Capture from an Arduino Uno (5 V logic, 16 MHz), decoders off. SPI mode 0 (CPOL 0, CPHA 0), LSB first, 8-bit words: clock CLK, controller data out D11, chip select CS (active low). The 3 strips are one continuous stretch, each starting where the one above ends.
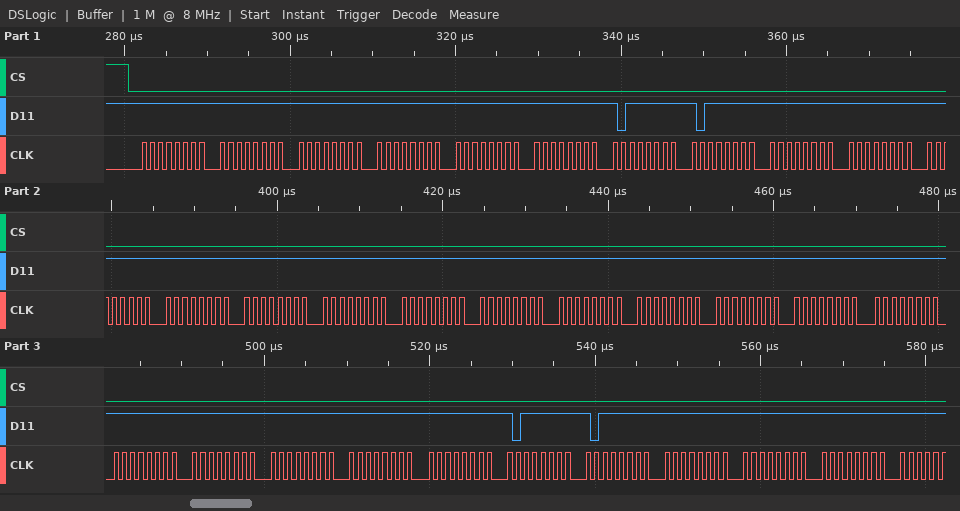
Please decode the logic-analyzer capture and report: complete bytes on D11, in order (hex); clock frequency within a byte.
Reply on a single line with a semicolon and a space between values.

FF FF FF FF FF FF FD FD FF FF FF FF FF FF FF FF FF FF FF FF FF FF FF FF FF FF FD FD FF FF FF; 1 MHz
